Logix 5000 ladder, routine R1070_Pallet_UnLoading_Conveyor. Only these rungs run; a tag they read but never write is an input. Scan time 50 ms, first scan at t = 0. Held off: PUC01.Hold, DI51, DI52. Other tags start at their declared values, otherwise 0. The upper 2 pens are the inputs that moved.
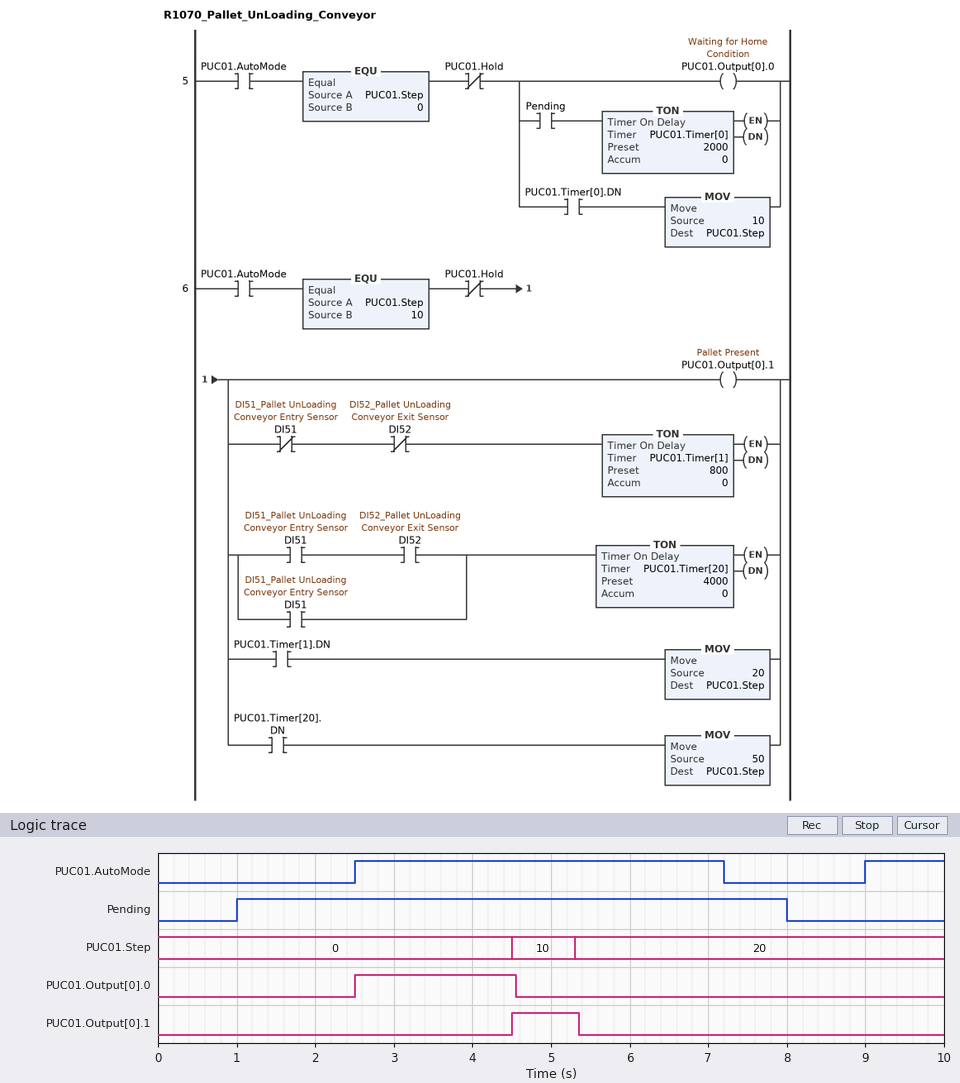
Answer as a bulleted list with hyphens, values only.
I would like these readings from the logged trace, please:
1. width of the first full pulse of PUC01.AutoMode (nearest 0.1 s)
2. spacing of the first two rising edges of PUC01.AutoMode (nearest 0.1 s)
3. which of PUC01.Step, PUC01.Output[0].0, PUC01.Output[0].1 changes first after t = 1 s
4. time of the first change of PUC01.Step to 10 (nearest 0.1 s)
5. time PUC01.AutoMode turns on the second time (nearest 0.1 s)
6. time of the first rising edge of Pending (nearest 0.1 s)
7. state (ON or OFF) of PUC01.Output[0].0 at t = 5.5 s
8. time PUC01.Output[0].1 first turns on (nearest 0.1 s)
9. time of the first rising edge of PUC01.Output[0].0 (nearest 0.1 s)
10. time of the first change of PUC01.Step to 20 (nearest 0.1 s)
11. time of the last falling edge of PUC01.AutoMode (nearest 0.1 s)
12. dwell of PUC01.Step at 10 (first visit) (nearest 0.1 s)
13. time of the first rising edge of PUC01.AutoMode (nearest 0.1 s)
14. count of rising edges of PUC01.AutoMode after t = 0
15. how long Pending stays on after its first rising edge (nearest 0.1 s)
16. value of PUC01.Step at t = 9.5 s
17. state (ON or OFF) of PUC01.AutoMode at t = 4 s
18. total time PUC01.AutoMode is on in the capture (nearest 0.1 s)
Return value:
- 4.7 s
- 6.5 s
- PUC01.Output[0].0
- 4.5 s
- 9.0 s
- 1.0 s
- OFF
- 4.5 s
- 2.5 s
- 5.3 s
- 7.2 s
- 0.8 s
- 2.5 s
- 2
- 7.0 s
- 20
- ON
- 5.7 s
